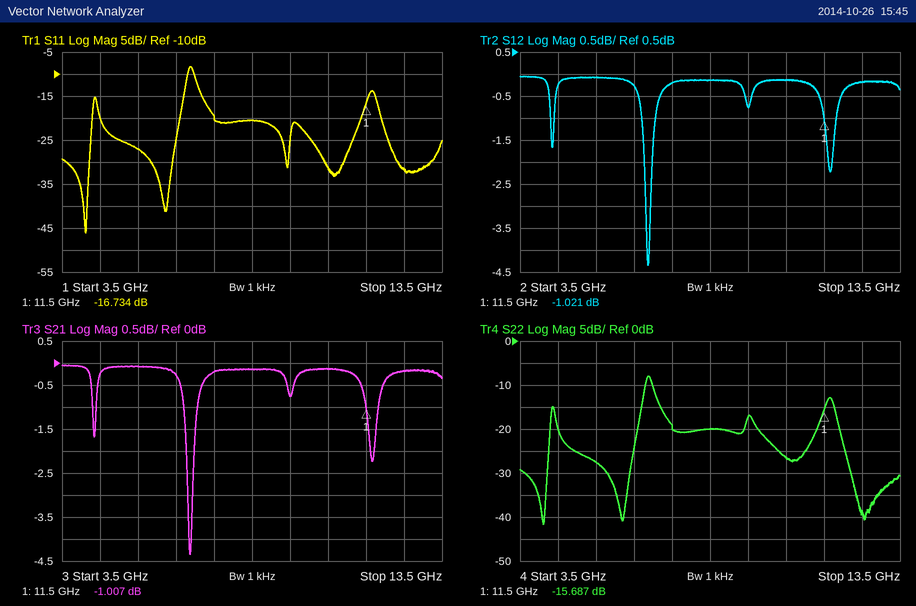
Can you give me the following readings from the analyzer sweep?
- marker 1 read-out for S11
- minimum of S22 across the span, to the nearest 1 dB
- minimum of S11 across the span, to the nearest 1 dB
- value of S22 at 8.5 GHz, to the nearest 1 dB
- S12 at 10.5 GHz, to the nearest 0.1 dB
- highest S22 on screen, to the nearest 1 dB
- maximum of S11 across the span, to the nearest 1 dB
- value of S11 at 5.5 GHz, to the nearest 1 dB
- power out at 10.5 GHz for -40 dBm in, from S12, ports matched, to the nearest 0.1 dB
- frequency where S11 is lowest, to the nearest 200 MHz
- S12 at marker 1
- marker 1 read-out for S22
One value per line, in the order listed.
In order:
-16.734 dB
-42 dB
-46 dB
-20 dB
-0.1 dB
-8 dB
-8 dB
-27 dB
-40.1 dBm
4.2 GHz
-1.021 dB
-15.687 dB
